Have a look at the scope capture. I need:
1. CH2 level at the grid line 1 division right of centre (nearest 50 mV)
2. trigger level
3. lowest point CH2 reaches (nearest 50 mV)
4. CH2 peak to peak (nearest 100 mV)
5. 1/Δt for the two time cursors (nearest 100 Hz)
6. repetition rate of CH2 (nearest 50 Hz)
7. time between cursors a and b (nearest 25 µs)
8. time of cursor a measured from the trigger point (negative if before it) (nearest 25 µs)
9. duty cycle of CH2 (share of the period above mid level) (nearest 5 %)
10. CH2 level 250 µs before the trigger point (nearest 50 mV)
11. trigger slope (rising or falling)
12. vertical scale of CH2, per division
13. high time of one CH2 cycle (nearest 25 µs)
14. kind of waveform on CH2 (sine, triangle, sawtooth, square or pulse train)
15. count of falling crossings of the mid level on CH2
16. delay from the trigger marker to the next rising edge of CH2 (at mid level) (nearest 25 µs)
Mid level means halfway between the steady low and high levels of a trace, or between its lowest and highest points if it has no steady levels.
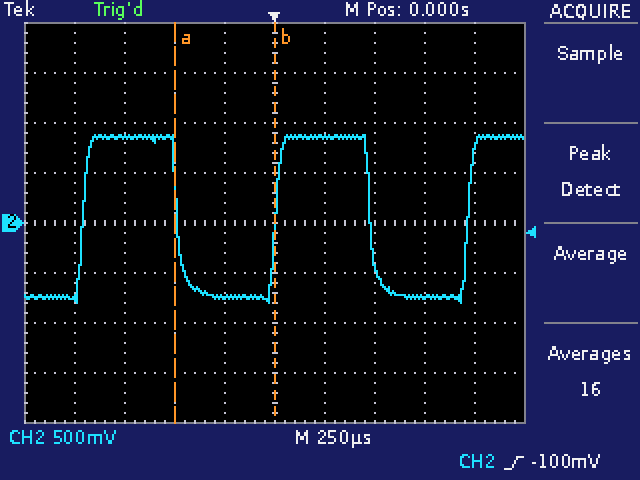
850 mV
-100 mV
-800 mV
1.70 V
2.0 kHz
1.05 kHz
500 µs
-500 µs
50 %
-750 mV
rising
500 mV
475 µs
square
2
975 µs
